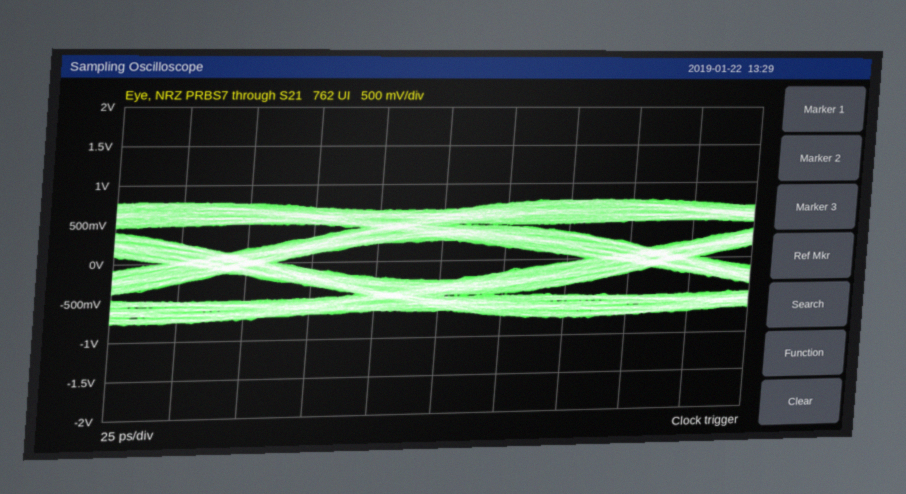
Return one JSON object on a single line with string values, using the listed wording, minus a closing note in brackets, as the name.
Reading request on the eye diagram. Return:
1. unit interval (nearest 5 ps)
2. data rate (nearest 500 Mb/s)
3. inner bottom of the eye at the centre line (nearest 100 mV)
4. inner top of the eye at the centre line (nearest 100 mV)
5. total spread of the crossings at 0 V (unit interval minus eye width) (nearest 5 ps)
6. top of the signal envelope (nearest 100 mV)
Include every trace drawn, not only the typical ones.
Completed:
{"unit interval": "165 ps", "data rate": "6.0 Gb/s", "inner bottom of the eye at the centre line": "-300 mV", "inner top of the eye at the centre line": "300 mV", "total spread of the crossings at 0 V (unit interval minus eye width)": "45 ps", "top of the signal envelope": "800 mV"}
